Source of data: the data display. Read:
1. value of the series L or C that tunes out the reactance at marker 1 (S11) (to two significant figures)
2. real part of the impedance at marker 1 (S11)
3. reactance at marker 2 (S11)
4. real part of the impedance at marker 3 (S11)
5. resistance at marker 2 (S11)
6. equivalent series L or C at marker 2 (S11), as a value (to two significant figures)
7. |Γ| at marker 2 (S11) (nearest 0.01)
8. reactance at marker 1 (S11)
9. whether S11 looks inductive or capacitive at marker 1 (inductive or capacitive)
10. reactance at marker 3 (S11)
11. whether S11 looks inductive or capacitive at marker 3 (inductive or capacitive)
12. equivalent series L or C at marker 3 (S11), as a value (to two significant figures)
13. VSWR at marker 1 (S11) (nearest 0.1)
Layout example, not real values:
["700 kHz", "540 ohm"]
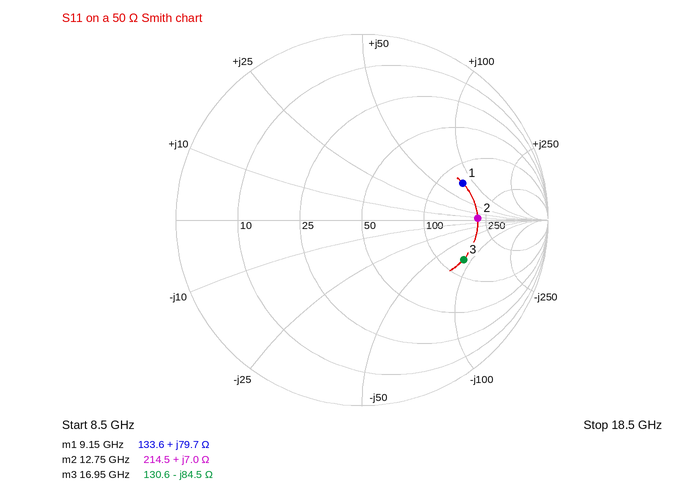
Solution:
["220 fF", "133.6 Ω", "+7.0 Ω", "130.6 Ω", "214.5 Ω", "87 pH", "0.62", "+79.7 Ω", "inductive", "-84.5 Ω", "capacitive", "110 fF", "3.7"]
